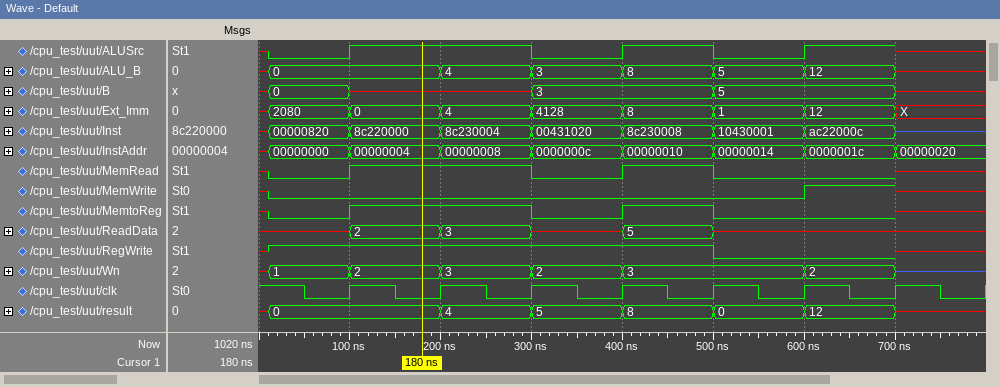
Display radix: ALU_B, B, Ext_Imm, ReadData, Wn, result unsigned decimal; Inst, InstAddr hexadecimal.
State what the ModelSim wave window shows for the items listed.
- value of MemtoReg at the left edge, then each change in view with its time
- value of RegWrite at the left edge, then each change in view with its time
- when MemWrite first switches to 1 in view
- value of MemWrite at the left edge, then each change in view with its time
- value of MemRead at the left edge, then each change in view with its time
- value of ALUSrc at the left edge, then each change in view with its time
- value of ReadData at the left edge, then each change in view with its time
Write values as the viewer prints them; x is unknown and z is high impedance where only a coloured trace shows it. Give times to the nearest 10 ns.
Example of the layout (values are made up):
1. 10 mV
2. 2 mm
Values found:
1. x, 0 at 10 ns, 1 at 100 ns, 0 at 300 ns, 1 at 400 ns, 0 at 500 ns, x at 700 ns
2. x, 1 at 10 ns, 0 at 500 ns, x at 700 ns
3. 600 ns
4. x, 0 at 10 ns, 1 at 600 ns, x at 700 ns
5. x, 0 at 10 ns, 1 at 100 ns, 0 at 300 ns, 1 at 400 ns, 0 at 500 ns, x at 700 ns
6. x, 0 at 10 ns, 1 at 100 ns, 0 at 300 ns, 1 at 400 ns, 0 at 500 ns, 1 at 600 ns, x at 700 ns
7. x, 2 at 100 ns, 3 at 200 ns, x at 300 ns, 5 at 400 ns, x at 500 ns
